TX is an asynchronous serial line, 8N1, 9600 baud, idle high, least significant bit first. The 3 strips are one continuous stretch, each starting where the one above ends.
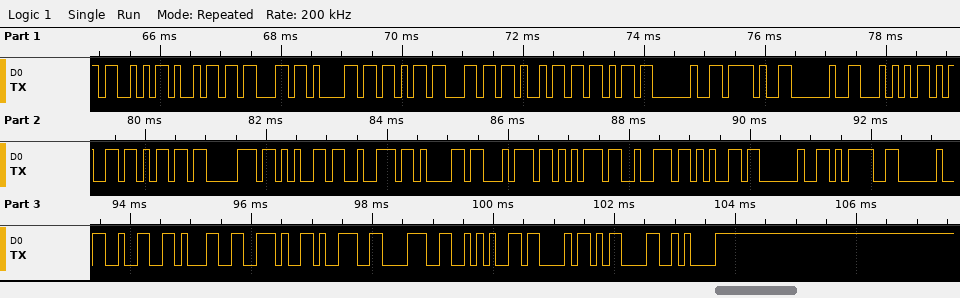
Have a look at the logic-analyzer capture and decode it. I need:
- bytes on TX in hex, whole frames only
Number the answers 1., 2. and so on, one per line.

1. 53 69 63 61 6B 6C 69 6B 20 2F 20 54 65 6D 70 65 72 61 74 75 72 65 20 3D 20 32 31 2E 39 38 2A 43 0D 0A
